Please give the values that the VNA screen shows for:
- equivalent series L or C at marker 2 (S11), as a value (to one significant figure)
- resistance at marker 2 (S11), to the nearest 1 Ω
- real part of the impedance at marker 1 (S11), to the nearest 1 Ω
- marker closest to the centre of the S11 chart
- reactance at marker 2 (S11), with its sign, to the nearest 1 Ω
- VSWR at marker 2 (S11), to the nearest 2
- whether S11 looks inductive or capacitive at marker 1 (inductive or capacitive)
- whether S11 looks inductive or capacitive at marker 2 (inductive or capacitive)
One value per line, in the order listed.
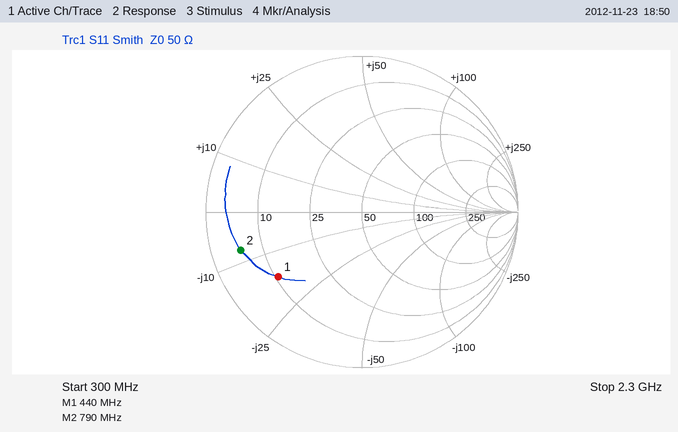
30 pF
5 Ω
11 Ω
marker 1
-8 Ω
10
capacitive
capacitive
